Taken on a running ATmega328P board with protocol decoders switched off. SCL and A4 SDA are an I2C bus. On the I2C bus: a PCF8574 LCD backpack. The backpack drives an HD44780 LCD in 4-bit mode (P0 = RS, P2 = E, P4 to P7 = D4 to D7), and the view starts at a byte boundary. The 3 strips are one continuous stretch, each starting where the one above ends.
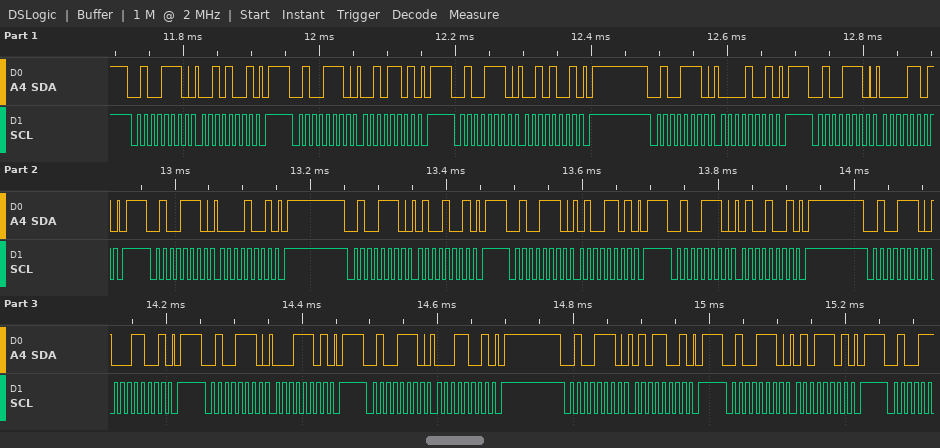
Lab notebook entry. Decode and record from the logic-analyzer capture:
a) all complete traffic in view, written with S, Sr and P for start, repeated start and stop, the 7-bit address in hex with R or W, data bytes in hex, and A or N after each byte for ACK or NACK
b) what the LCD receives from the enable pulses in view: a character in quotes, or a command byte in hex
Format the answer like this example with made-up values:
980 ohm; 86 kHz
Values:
S 27W A 29 A P S 27W A 2D A P S 27W A 29 A P S 27W A 09 A P S 27W A 0D A P S 27W A 09 A P S 27W A 49 A P S 27W A 4D A P S 27W A 49 A P S 27W A 19 A P S 27W A 1D A P S 27W A 19 A P S 27W A 59 A P S 27W A 5D A P; ' ' 'A'
